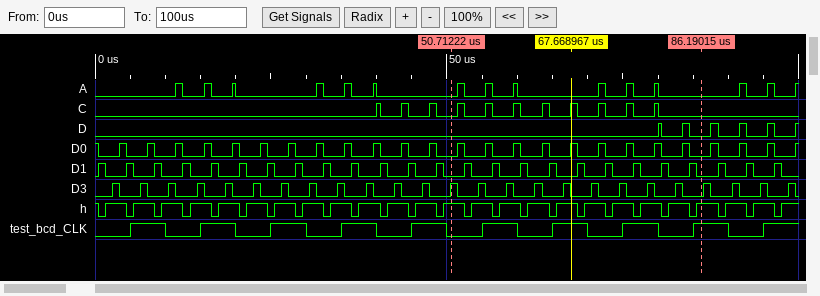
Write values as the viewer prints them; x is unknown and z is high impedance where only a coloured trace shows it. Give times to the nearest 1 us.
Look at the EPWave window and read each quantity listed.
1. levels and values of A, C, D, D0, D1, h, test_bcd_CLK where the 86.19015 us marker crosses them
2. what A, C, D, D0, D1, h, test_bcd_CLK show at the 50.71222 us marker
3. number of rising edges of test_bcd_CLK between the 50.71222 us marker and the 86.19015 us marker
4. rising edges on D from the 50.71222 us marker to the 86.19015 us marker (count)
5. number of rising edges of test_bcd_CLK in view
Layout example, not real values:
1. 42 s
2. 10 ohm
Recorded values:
1. A=0, C=0, D=0, D0=0, D1=0, h=1, test_bcd_CLK=1
2. A=0, C=0, D=0, D0=0, D1=0, h=1, test_bcd_CLK=0
3. 4
4. 2
5. 10
